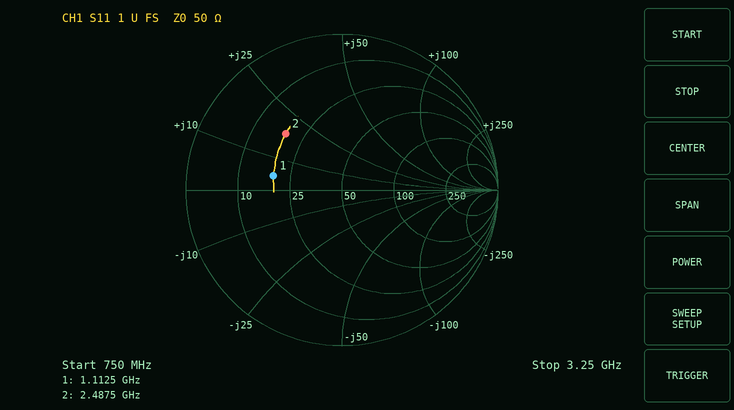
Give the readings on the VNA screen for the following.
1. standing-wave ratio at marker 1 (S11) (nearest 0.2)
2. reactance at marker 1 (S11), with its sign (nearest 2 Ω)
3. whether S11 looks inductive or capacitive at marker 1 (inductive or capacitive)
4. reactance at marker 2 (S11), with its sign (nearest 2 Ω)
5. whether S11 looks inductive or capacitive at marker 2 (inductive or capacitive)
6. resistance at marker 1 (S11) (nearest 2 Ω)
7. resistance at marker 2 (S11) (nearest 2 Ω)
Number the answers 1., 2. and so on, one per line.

1. 2.6
2. +4 Ω
3. inductive
4. +18 Ω
5. inductive
6. 20 Ω
7. 18 Ω
